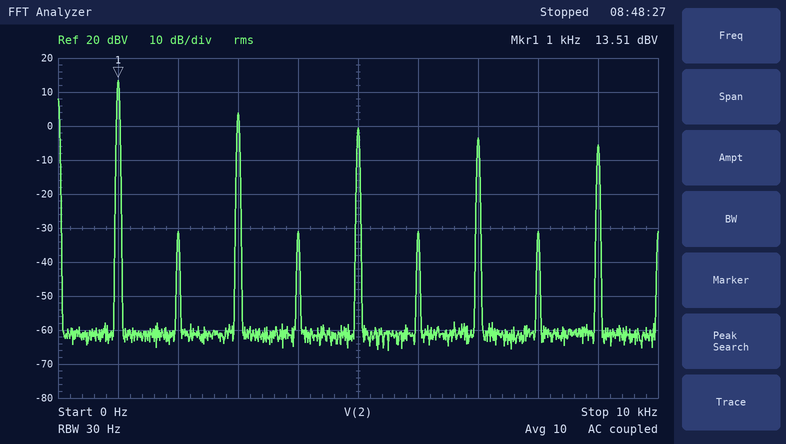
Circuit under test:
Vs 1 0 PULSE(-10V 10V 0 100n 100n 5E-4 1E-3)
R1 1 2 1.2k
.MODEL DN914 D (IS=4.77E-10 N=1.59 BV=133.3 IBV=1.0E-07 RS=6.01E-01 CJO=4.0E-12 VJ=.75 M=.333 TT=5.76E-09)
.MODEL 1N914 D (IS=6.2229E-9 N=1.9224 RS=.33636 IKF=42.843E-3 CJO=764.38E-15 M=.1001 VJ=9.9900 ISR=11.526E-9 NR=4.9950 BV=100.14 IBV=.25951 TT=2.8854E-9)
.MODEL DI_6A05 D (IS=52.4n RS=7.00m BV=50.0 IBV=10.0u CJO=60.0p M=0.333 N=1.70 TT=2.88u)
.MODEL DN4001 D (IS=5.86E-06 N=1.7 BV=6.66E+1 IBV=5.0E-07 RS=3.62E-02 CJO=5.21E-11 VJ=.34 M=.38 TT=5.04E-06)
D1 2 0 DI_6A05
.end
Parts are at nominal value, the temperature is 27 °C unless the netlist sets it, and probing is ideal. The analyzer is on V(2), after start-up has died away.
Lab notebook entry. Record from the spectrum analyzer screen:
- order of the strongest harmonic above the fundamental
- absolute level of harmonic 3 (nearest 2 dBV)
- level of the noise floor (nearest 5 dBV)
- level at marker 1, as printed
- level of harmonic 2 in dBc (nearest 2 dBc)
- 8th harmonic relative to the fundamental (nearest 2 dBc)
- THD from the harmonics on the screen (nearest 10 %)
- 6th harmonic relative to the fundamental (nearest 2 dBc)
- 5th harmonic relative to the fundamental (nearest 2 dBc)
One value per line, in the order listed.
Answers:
3
4 dBV
-60 dBV
13.51 dBV
-44 dBc
-44 dBc
40 %
-44 dBc
-14 dBc
